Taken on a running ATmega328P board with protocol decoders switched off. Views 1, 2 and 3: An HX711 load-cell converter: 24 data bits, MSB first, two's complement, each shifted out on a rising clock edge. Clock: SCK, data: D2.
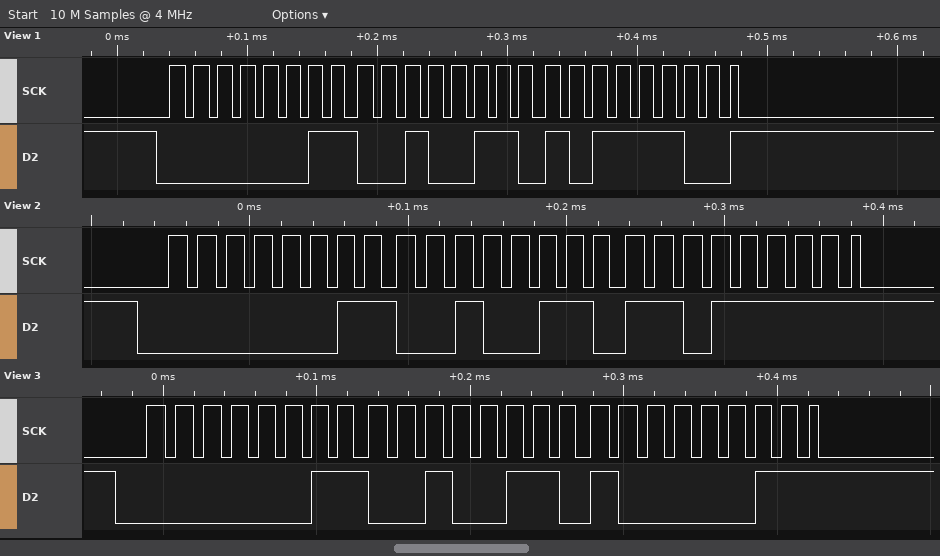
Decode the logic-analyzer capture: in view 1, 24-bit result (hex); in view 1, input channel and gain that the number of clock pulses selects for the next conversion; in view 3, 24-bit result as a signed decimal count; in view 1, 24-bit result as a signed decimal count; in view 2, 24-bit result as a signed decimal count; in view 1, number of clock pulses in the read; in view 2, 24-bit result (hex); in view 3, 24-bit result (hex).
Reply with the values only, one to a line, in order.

0x0326BC
channel A, gain 128
206467
206524
206559
25
0x0326DF
0x032683
